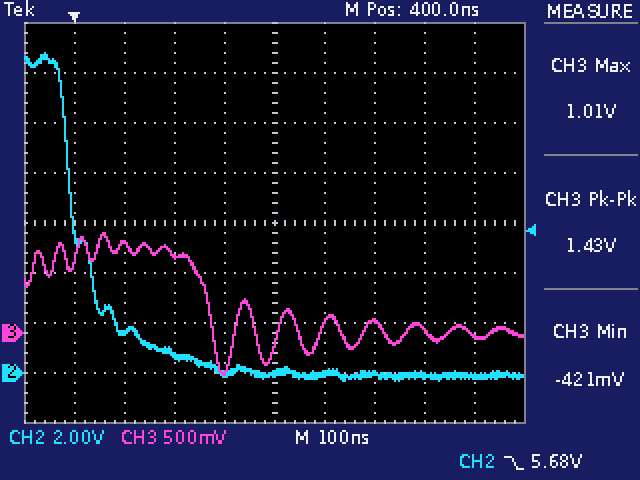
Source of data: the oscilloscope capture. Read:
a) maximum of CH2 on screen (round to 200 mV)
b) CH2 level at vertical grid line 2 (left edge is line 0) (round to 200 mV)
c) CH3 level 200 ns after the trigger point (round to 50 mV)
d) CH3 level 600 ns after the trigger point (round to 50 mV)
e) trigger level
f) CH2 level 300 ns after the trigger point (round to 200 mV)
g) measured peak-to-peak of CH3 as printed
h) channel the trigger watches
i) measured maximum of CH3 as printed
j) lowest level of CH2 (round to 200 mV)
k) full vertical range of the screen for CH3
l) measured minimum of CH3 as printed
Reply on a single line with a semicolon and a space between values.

12.8 V; 1.6 V; 800 mV; 100 mV; 5.68 V; 0.0 V; 1.43 V; CH2; 1.01 V; -400 mV; 4 V; -421 mV
